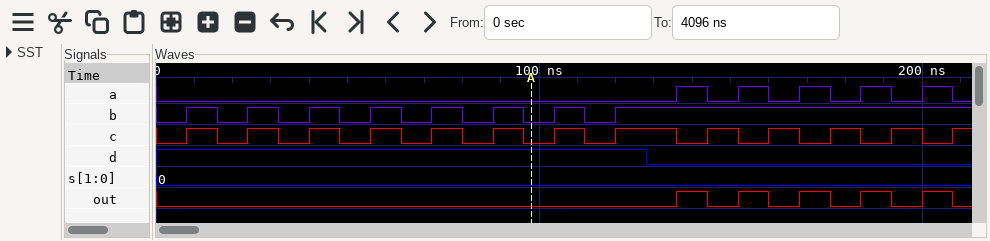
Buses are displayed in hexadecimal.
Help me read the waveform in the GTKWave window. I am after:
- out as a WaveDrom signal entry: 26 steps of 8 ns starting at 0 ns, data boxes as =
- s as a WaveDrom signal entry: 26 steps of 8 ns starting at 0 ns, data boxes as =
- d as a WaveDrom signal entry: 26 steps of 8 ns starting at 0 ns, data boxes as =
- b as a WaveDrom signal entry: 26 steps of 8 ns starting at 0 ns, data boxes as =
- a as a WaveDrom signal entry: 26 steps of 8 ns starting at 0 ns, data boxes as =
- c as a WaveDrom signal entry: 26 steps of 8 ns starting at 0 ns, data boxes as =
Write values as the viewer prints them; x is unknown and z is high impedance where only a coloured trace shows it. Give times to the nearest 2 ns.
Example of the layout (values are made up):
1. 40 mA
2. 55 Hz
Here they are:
1. {name: 'out', wave: '0................101010101'}
2. {name: 's', wave: '=.........................', data: '0'}
3. {name: 'd', wave: '1...............0.........'}
4. {name: 'b', wave: '0101010101010101..........'}
5. {name: 'a', wave: '0................101010101'}
6. {name: 'c', wave: '0101010101010101.010101010'}
